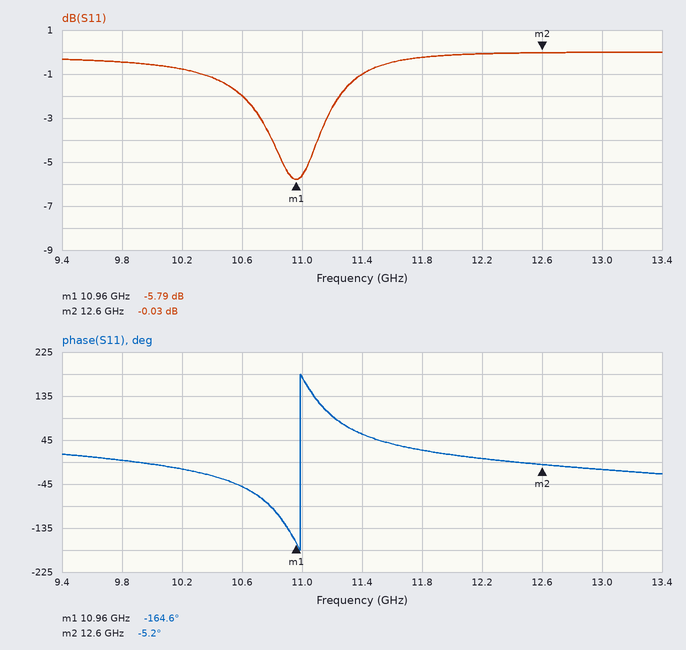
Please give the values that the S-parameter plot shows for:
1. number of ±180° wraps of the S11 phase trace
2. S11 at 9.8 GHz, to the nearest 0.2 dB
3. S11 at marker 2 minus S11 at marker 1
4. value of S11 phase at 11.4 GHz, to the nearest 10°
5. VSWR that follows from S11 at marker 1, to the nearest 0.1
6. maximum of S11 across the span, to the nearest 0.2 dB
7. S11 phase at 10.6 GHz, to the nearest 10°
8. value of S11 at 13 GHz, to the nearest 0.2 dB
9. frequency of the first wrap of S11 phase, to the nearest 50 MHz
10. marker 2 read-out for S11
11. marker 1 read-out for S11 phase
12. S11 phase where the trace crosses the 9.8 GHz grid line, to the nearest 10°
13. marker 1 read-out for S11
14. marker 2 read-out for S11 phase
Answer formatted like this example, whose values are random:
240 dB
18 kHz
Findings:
1
-0.4 dB
5.76 dB
60°
3.1
0.0 dB
-50°
0.0 dB
11.00 GHz
-0.03 dB
-164.6°
0°
-5.79 dB
-5.2°
